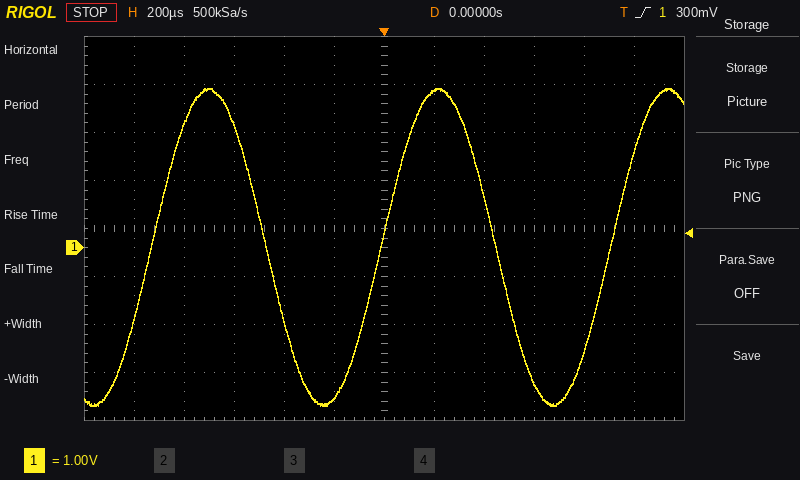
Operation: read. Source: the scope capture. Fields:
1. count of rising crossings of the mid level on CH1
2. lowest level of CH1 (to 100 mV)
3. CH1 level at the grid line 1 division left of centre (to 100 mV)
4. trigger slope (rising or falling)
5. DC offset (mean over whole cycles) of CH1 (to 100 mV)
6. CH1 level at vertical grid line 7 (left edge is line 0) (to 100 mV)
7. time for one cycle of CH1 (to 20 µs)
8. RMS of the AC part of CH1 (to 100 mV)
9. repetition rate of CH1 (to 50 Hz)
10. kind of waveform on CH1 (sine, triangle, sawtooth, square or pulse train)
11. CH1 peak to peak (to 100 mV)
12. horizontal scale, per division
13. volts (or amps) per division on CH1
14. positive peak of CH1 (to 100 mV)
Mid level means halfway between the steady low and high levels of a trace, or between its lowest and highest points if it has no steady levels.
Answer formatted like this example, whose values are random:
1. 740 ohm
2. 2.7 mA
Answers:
1. 3
2. -3.3 V
3. -3.1 V
4. rising
5. 0.0 V
6. 3.3 V
7. 920 µs
8. 2.3 V
9. 1.10 kHz
10. sine
11. 6.6 V
12. 200 µs
13. 1 V
14. 3.3 V
